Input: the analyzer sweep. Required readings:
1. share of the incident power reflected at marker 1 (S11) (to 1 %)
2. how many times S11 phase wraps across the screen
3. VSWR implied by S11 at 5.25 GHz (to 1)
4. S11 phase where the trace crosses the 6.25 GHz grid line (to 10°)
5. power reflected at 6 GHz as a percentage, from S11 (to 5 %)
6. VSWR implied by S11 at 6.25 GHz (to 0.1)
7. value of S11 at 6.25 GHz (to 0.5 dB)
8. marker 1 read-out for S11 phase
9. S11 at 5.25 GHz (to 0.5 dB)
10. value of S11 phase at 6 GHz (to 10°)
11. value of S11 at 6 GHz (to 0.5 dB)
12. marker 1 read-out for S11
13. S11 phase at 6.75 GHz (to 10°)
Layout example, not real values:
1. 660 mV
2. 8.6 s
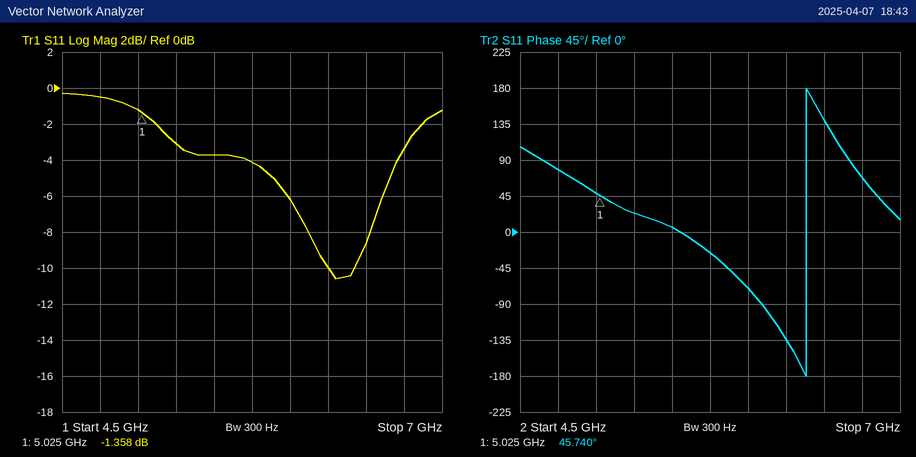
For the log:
1. 73 %
2. 1
3. 6
4. -130°
5. 25 %
6. 1.9
7. -10.0 dB
8. 45.740°
9. -3.0 dB
10. -70°
11. -6.0 dB
12. -1.358 dB
13. 70°
